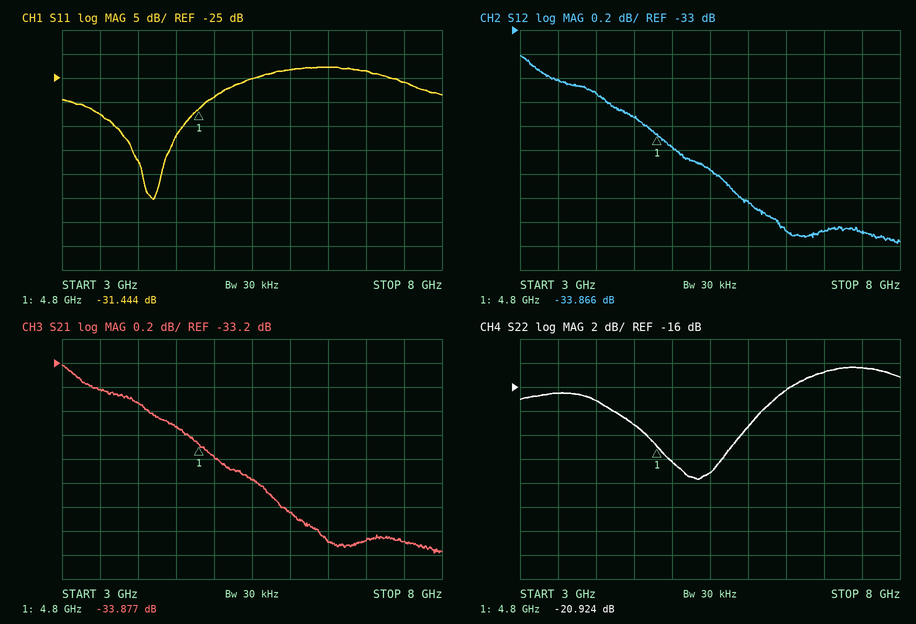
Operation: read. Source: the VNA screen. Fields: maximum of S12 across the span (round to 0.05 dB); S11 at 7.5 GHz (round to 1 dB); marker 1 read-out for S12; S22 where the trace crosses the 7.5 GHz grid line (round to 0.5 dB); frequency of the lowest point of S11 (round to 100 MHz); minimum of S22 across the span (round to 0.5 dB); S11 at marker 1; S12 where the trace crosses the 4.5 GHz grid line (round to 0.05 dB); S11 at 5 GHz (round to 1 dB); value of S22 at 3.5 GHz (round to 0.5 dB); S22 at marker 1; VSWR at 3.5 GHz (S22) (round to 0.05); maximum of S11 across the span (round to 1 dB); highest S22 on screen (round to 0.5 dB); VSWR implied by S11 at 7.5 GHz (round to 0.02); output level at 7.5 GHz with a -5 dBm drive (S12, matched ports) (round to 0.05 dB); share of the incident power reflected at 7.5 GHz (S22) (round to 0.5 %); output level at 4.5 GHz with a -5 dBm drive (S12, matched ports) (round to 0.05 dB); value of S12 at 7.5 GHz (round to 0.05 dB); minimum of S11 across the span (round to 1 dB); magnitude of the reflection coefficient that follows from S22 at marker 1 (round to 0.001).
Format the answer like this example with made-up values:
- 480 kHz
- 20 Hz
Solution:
- -33.20 dB
- -26 dB
- -33.866 dB
- -14.5 dB
- 4.2 GHz
- -23.5 dB
- -31.444 dB
- -33.75 dB
- -29 dB
- -16.5 dB
- -20.924 dB
- 1.35
- -23 dB
- -14.5 dB
- 1.10
- -39.70 dBm
- 3.5 %
- -38.75 dBm
- -34.70 dB
- -50 dB
- 0.090
